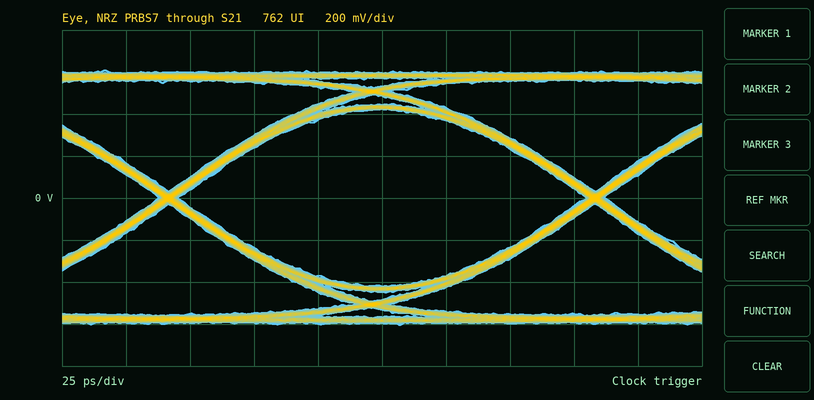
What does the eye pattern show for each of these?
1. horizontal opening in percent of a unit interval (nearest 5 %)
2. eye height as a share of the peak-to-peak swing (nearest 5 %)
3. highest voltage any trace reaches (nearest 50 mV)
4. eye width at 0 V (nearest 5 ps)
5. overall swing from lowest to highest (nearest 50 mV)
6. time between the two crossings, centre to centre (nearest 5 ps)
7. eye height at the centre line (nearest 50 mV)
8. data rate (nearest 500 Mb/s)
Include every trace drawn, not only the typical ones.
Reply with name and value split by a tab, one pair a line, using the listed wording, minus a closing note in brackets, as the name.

horizontal opening in percent of a unit interval	95 %
eye height as a share of the peak-to-peak swing	70 %
highest voltage any trace reaches	600 mV
eye width at 0 V	160 ps
overall swing from lowest to highest	1.20 V
time between the two crossings, centre to centre	165 ps
eye height at the centre line	850 mV
data rate	6.0 Gb/s
